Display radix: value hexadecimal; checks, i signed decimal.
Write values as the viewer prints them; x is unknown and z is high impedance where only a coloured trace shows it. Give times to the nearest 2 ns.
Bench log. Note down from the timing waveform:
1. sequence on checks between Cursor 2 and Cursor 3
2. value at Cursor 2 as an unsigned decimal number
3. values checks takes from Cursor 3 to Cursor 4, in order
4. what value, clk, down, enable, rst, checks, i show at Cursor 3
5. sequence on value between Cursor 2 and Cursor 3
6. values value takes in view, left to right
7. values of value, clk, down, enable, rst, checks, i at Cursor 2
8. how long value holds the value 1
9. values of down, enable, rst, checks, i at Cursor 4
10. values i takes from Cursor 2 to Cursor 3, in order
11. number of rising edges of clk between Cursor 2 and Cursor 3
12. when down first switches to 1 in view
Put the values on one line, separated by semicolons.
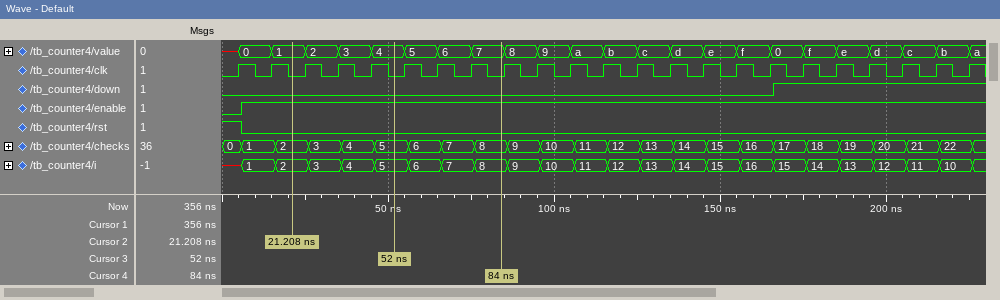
2, 3, 4, 5; 1; 5, 6, 7, 8; value=4, clk=0, down=0, enable=1, rst=0, checks=5, i=5; 1, 2, 3, 4; x, 0, 1, 2, 3, 4, 5, 6, 7, 8, 9, a, b, c, d, e, f, 0, f, e, d, c, b, a; value=1, clk=0, down=0, enable=1, rst=0, checks=2, i=2; 10 ns; down=0, enable=1, rst=0, checks=8, i=8; 2, 3, 4, 5; 3; 166 ns
